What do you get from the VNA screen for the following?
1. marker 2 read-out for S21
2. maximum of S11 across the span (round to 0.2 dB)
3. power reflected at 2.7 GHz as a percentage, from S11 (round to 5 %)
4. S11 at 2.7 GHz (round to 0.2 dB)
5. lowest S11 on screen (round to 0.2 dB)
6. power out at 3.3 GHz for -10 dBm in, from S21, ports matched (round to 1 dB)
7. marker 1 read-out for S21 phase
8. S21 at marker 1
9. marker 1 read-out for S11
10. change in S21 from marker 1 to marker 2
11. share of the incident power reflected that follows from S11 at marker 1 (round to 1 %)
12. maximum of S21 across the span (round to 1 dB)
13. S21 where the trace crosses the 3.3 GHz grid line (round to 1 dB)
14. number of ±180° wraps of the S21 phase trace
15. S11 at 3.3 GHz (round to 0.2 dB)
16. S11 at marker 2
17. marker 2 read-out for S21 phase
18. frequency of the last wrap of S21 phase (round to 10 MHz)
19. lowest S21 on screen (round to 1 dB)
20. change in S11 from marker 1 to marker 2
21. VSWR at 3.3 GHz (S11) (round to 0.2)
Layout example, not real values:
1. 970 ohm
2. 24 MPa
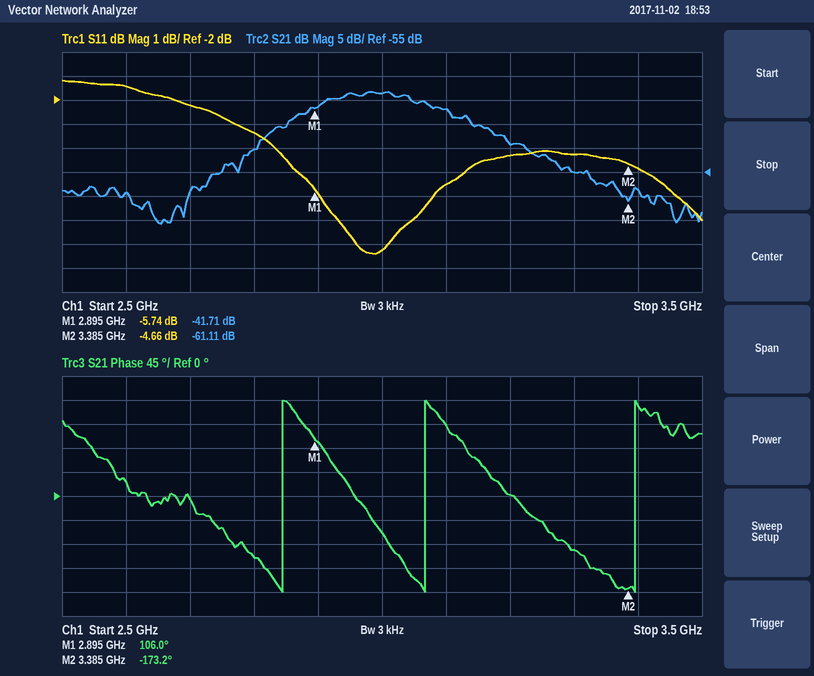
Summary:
1. -61.11 dB
2. -1.2 dB
3. 60 %
4. -2.2 dB
5. -8.4 dB
6. -65 dBm
7. 106.0°
8. -41.71 dB
9. -5.74 dB
10. -19.40 dB
11. 27 %
12. -38 dB
13. -55 dB
14. 3
15. -4.2 dB
16. -4.66 dB
17. -173.2°
18. 3.40 GHz
19. -66 dB
20. 1.08 dB
21. 4.2
